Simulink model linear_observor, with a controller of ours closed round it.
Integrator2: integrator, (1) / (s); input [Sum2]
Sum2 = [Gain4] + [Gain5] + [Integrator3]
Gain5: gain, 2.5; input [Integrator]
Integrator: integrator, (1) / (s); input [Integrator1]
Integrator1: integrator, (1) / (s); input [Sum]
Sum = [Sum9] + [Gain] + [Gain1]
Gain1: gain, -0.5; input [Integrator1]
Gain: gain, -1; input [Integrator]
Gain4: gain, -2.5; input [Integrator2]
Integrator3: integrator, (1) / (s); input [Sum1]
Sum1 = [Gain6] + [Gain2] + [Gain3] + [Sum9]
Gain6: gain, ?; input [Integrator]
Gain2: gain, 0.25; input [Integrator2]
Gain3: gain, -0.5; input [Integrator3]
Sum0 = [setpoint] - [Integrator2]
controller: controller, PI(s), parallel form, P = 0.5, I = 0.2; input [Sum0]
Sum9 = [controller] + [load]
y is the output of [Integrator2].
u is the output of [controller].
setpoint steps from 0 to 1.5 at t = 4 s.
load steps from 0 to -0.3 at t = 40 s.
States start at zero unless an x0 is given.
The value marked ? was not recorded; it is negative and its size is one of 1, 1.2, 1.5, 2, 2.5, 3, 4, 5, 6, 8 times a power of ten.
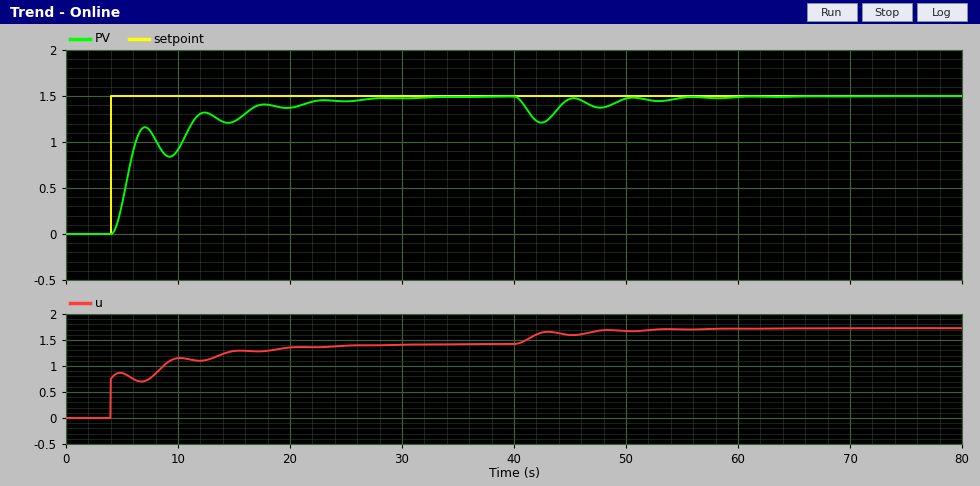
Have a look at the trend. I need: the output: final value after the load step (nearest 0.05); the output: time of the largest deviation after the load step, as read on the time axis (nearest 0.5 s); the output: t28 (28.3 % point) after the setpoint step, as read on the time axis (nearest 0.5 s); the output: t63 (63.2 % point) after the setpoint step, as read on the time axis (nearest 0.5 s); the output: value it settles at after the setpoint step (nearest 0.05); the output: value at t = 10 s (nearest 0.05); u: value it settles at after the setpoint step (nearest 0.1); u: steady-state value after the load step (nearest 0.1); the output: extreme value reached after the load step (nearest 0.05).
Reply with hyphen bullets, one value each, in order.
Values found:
- 1.50
- 42.5 s
- 5.0 s
- 6.0 s
- 1.50
- 0.90
- 1.4
- 1.7
- 1.20
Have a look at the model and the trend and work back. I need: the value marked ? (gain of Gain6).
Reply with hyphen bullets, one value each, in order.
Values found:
- -1.2
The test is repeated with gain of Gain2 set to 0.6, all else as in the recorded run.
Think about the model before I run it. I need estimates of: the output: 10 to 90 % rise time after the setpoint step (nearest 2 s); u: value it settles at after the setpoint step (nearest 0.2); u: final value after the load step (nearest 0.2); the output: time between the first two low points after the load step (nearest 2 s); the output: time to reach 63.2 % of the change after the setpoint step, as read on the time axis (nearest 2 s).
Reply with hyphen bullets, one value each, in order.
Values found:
- 6 s
- 1.0
- 1.2
- 6 s
- 6 s
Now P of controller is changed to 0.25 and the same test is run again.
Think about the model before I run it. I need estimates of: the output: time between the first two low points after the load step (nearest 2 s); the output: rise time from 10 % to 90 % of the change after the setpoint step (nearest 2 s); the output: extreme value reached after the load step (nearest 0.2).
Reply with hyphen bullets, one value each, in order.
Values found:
- 6 s
- 8 s
- 1.2
